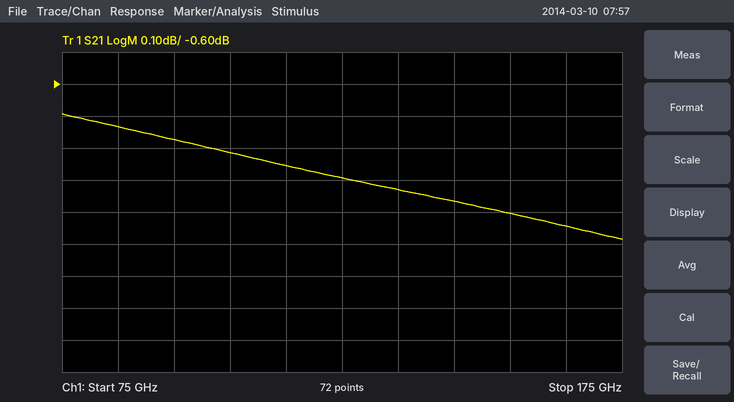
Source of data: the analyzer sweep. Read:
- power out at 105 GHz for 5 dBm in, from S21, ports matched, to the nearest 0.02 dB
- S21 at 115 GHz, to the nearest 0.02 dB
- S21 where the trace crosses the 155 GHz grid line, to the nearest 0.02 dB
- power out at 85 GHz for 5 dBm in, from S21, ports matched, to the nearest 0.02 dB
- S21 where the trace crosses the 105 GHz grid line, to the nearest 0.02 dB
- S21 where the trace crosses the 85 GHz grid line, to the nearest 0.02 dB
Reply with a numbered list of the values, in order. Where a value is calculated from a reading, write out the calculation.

1. 5 dBm + (-0.82 dB) = 4.18 dBm
2. -0.86 dB
3. -1.00 dB
4. 5 dBm + (-0.74 dB) = 4.26 dBm
5. -0.82 dB
6. -0.74 dB
